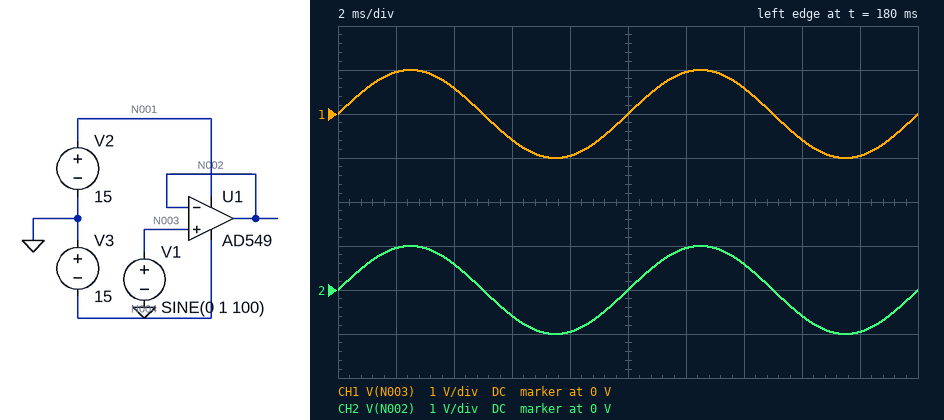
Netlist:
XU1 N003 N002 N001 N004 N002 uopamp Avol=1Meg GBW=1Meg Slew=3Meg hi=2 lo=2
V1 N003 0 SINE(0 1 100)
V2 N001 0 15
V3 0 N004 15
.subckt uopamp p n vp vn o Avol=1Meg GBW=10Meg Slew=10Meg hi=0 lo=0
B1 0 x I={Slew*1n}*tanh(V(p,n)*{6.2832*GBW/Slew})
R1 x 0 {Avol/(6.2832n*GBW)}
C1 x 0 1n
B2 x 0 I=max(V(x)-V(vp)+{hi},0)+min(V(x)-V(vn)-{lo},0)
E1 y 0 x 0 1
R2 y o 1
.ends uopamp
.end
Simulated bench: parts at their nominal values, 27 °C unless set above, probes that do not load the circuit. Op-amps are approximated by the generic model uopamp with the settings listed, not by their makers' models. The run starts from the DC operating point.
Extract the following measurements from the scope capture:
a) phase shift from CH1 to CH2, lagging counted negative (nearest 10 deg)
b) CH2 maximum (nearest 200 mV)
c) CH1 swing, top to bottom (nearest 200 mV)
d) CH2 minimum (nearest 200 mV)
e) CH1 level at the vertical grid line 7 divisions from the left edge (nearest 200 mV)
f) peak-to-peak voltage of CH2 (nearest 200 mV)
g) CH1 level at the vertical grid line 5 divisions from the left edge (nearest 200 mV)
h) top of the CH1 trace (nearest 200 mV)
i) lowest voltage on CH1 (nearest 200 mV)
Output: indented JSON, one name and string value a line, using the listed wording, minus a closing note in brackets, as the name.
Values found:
{
  "phase shift from CH1 to CH2, lagging counted negative": "0 deg",
  "CH2 maximum": "1.0 V",
  "CH1 swing, top to bottom": "2.0 V",
  "CH2 minimum": "-1.0 V",
  "CH1 level at the vertical grid line 7 divisions from the left edge": "600 mV",
  "peak-to-peak voltage of CH2": "2.0 V",
  "CH1 level at the vertical grid line 5 divisions from the left edge": "0 V",
  "top of the CH1 trace": "1.0 V",
  "lowest voltage on CH1": "-1.0 V"
}
